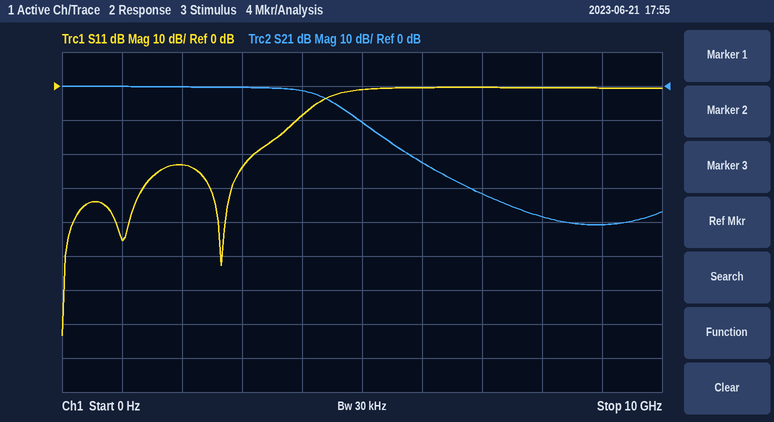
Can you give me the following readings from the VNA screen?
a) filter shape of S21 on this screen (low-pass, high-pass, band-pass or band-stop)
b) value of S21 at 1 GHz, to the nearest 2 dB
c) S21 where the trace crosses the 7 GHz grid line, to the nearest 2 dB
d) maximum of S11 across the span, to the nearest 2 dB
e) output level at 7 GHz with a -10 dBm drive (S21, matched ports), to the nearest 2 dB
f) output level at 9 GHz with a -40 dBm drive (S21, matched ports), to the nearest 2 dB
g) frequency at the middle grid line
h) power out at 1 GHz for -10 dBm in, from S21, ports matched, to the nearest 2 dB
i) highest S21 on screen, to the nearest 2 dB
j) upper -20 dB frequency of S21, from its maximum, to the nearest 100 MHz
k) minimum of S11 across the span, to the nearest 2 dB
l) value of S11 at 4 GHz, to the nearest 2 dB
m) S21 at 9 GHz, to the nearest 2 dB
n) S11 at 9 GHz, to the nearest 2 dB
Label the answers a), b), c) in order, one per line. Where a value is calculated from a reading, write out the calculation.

a) low-pass
b) 0 dB
c) -32 dB
d) 0 dB
e) -10 dBm + (-32 dB) = -42 dBm
f) -40 dBm + (-40 dB) = -80 dBm
g) 5 GHz
h) -10 dBm + (0 dB) = -10 dBm
i) 0 dB
j) 5.8 GHz
k) -74 dB
l) -8 dB
m) -40 dB
n) 0 dB
